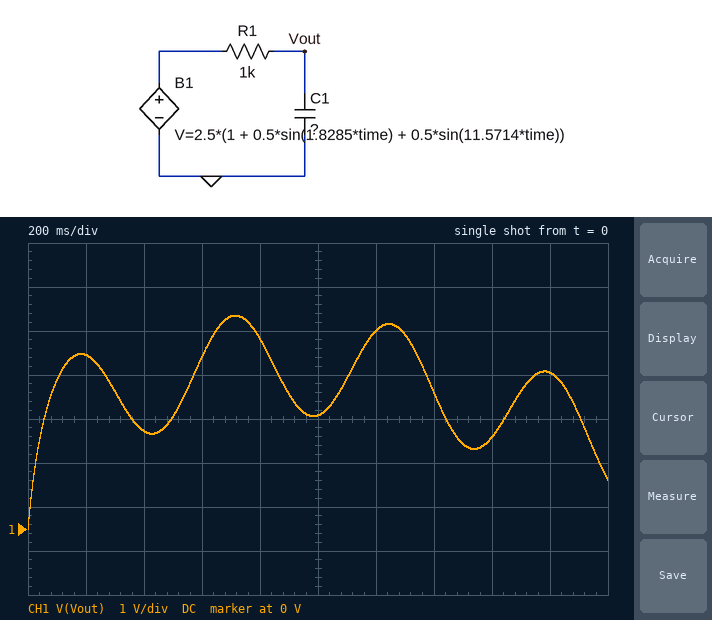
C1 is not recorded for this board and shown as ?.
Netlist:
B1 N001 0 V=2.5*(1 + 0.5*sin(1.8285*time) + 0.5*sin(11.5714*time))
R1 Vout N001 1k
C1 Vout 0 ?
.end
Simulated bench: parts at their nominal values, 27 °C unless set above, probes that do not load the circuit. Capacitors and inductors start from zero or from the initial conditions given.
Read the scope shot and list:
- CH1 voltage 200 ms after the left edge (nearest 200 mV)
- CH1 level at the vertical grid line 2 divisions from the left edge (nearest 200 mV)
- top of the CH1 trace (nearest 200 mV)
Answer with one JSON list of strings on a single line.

["4.0 V", "2.2 V", "4.8 V"]
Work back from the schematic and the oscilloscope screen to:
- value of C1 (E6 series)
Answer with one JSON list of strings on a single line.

["33 µF"]
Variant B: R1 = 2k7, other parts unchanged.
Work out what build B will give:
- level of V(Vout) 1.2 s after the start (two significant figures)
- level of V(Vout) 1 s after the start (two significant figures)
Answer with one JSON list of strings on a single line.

["4.0 V", "2.9 V"]
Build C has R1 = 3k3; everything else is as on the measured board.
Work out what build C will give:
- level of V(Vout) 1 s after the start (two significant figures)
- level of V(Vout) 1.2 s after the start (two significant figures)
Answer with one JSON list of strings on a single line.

["3.0 V", "3.9 V"]
